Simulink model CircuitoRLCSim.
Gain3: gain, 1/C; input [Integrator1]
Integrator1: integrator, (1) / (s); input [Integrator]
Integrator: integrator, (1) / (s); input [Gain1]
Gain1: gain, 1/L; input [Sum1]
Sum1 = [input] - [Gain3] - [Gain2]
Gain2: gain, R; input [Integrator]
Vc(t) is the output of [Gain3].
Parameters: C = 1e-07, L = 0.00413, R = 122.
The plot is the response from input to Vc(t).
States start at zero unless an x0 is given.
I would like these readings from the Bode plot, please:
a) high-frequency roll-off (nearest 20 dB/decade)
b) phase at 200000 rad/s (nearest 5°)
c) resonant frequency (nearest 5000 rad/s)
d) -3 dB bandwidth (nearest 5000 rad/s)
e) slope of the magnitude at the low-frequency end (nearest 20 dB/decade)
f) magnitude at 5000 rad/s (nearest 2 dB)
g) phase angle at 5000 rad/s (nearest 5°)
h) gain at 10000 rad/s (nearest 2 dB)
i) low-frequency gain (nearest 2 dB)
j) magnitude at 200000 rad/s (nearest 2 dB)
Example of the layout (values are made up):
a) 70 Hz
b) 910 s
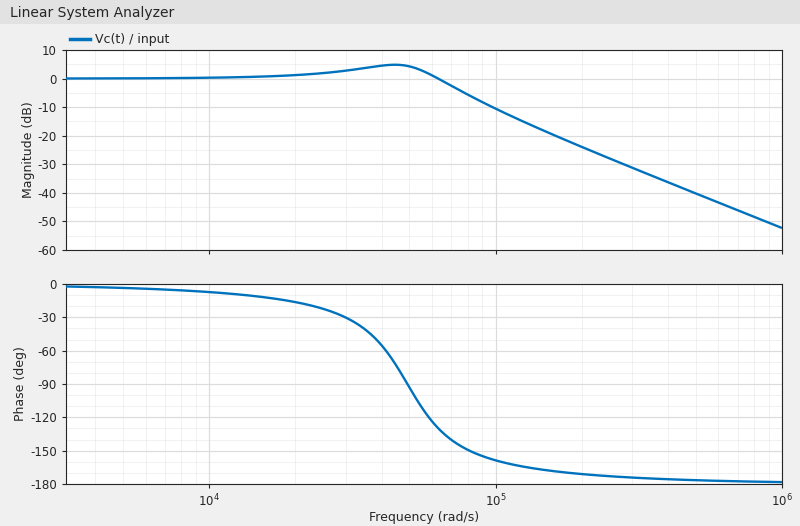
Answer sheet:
a) -40 dB/decade
b) -170°
c) 45000 rad/s
d) 70000 rad/s
e) 0 dB/decade
f) 0 dB
g) -5°
h) 0 dB
i) 0 dB
j) -24 dB
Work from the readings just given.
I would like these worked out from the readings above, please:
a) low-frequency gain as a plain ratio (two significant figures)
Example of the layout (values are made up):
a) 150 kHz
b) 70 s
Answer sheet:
a) 1.0
